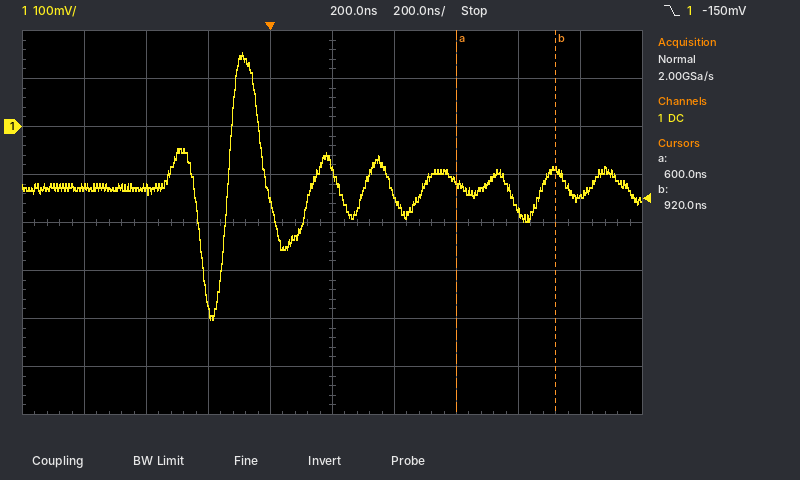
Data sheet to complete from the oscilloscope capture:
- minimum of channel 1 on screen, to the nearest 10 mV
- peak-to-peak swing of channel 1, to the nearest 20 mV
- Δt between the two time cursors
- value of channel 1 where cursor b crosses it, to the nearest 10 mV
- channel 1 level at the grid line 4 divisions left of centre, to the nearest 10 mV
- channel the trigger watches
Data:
-400 mV
560 mV
320 ns
-90 mV
-130 mV
channel 1
